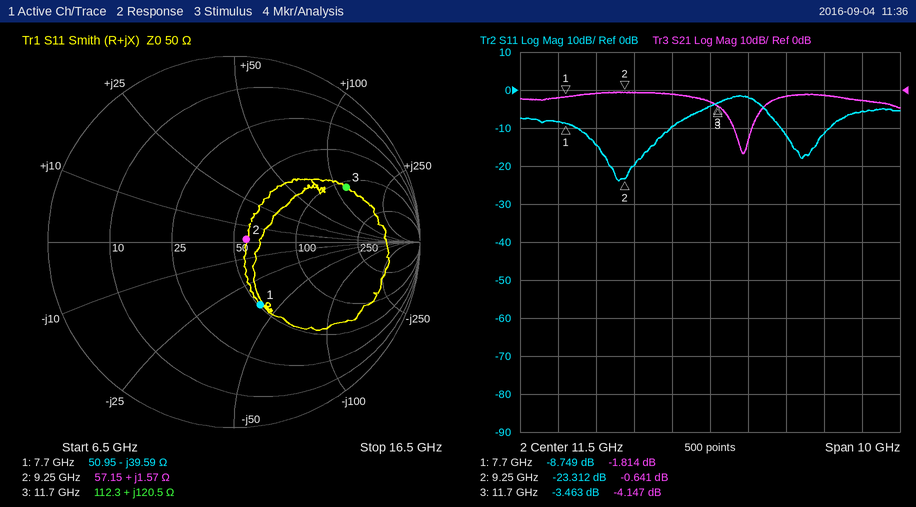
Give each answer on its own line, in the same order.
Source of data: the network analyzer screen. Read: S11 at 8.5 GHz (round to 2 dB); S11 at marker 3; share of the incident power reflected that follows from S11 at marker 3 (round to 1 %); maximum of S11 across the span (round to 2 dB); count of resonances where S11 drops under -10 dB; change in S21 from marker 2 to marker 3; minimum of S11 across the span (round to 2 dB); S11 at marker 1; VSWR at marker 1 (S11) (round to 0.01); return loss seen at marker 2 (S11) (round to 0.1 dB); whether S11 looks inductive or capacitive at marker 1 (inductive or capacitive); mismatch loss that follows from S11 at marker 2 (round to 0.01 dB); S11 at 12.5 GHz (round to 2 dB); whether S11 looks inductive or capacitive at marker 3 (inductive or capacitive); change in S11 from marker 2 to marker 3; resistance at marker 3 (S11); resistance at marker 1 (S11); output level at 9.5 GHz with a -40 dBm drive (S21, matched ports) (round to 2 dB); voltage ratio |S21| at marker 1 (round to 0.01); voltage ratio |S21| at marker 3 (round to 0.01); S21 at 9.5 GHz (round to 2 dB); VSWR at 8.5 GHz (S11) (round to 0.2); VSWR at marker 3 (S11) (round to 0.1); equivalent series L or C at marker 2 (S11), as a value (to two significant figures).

-14 dB
-3.463 dB
45 %
-2 dB
2
-3.506 dB
-24 dB
-8.749 dB
2.15
23.3 dB
capacitive
0.02 dB
-2 dB
inductive
19.849 dB
112.3 Ω
50.95 Ω
-40 dBm
0.81
0.62
0 dB
1.4
5.1
27 pH
